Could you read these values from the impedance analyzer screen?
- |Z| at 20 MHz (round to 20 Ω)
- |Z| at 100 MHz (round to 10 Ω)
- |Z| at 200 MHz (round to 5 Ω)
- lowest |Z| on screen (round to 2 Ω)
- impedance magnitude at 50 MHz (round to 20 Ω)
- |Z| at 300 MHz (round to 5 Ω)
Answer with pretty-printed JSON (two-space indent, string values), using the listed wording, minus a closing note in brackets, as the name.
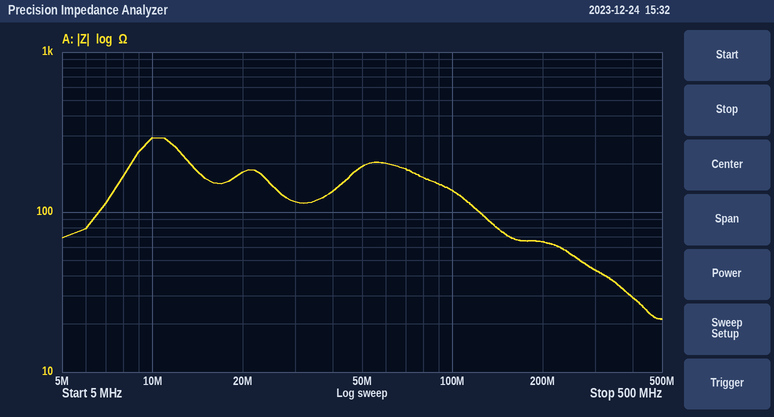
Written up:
{
  "|Z| at 20 MHz": "180 Ω",
  "|Z| at 100 MHz": "140 Ω",
  "|Z| at 200 MHz": "65 Ω",
  "lowest |Z| on screen": "22 Ω",
  "impedance magnitude at 50 MHz": "200 Ω",
  "|Z| at 300 MHz": "45 Ω"
}
